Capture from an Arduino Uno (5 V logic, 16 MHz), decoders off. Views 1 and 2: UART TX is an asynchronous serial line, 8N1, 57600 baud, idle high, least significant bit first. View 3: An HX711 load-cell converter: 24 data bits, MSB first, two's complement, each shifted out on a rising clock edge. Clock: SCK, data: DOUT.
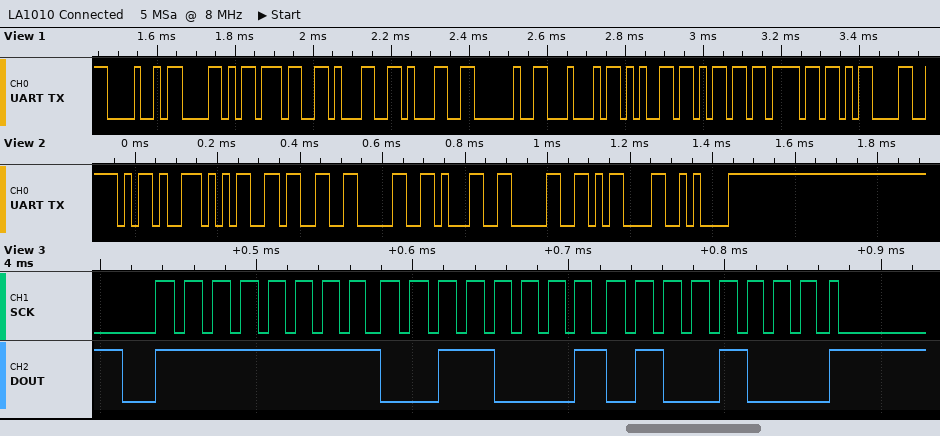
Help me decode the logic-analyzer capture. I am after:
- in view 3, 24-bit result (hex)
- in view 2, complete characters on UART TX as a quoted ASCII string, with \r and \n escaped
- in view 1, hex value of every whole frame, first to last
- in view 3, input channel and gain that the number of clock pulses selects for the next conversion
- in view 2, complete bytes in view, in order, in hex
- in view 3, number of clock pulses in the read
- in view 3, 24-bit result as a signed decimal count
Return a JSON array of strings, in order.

["0xFF3148", "\"-53010\\r\\n\"", "0x48 0x58 0x37 0x31 0x31 0x20 0x44 0x65 0x6D 0x6F 0x0D", "channel A, gain 128", "2D 35 33 30 31 30 0D 0A", "25", "-52920"]
